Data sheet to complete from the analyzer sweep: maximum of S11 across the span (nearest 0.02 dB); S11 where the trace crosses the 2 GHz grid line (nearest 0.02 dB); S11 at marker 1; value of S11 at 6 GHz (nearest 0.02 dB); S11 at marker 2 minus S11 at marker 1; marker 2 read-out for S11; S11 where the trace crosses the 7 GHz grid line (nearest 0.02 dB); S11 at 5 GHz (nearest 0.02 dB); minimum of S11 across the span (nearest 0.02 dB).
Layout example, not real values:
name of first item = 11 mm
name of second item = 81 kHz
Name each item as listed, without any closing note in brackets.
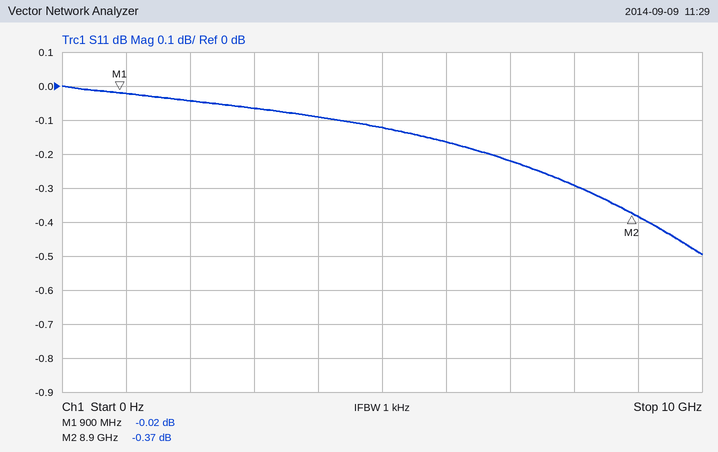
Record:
maximum of S11 across the span = 0.00 dB
S11 where the trace crosses the 2 GHz grid line = -0.04 dB
S11 at marker 1 = -0.02 dB
value of S11 at 6 GHz = -0.16 dB
S11 at marker 2 minus S11 at marker 1 = -0.35 dB
marker 2 read-out for S11 = -0.37 dB
S11 where the trace crosses the 7 GHz grid line = -0.22 dB
S11 at 5 GHz = -0.12 dB
minimum of S11 across the span = -0.50 dB
